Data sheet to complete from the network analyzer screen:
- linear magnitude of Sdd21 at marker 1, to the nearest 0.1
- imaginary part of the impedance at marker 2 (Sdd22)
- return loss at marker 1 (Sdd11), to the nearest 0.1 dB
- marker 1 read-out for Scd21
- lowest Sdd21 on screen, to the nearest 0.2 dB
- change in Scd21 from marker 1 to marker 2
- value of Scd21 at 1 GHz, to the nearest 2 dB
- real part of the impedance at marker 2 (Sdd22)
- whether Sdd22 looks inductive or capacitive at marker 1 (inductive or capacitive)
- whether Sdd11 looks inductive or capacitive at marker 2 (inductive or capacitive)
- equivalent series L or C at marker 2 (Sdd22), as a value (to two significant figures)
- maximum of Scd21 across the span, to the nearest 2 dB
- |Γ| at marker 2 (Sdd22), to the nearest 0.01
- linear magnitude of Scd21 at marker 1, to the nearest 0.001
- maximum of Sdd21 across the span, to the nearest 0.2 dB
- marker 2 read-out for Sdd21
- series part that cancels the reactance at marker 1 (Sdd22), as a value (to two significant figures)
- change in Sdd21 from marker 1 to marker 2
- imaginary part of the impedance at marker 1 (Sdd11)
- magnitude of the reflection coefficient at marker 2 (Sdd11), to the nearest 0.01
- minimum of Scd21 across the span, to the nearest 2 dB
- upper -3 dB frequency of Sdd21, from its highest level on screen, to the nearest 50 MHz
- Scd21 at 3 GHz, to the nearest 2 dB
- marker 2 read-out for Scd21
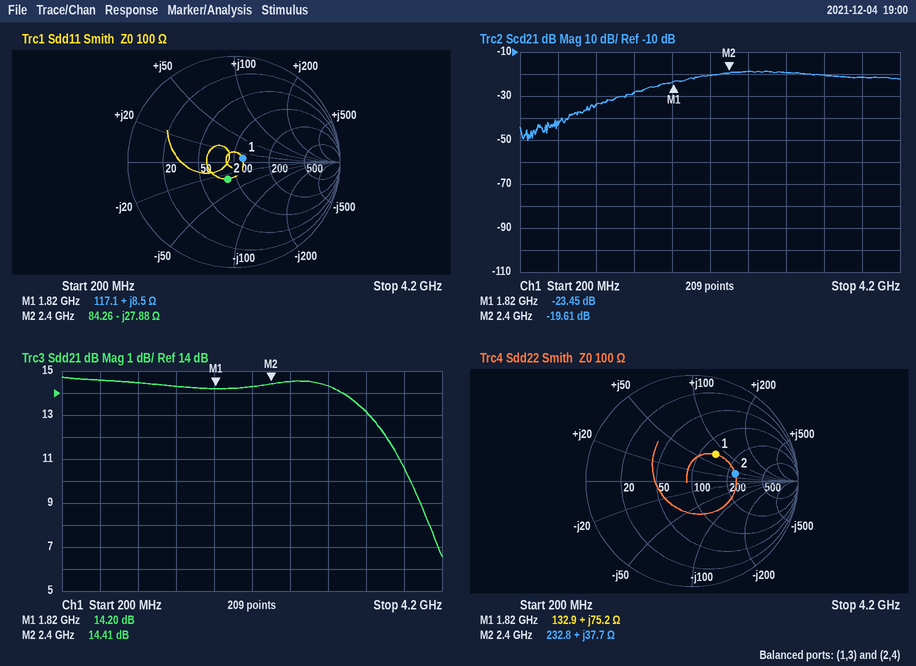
5.1
+37.7 Ω
21.1 dB
-23.45 dB
6.6 dB
3.84 dB
-34 dB
232.8 Ω
inductive
capacitive
2.5 nH
-18 dB
0.41
0.067
14.8 dB
14.41 dB
1.2 pF
0.21 dB
+8.5 Ω
0.17
-50 dB
3.65 GHz
-20 dB
-19.61 dB
